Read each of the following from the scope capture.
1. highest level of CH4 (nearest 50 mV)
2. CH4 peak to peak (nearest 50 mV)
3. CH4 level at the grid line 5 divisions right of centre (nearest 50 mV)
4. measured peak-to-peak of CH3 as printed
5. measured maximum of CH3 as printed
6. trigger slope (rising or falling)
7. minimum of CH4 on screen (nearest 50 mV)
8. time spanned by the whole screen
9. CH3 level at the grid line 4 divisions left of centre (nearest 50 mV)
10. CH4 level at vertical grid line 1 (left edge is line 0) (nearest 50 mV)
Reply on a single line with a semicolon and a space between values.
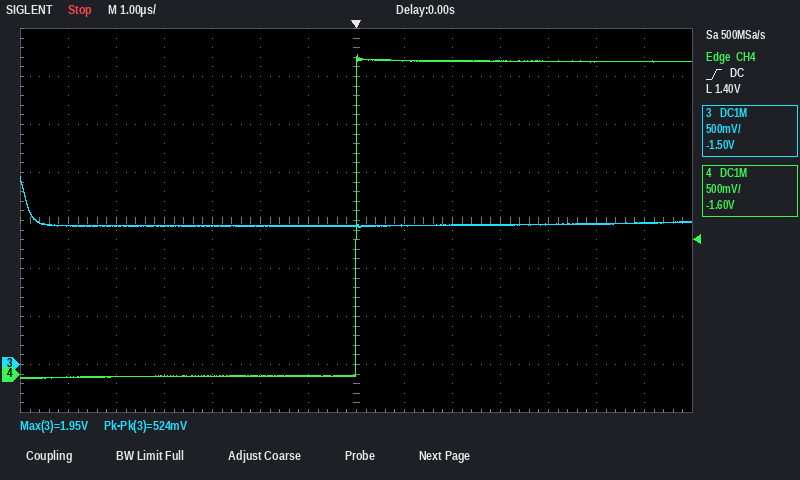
3.35 V; 3.40 V; 3.25 V; 524 mV; 1.95 V; rising; -50 mV; 14 µs; 1.45 V; -50 mV
